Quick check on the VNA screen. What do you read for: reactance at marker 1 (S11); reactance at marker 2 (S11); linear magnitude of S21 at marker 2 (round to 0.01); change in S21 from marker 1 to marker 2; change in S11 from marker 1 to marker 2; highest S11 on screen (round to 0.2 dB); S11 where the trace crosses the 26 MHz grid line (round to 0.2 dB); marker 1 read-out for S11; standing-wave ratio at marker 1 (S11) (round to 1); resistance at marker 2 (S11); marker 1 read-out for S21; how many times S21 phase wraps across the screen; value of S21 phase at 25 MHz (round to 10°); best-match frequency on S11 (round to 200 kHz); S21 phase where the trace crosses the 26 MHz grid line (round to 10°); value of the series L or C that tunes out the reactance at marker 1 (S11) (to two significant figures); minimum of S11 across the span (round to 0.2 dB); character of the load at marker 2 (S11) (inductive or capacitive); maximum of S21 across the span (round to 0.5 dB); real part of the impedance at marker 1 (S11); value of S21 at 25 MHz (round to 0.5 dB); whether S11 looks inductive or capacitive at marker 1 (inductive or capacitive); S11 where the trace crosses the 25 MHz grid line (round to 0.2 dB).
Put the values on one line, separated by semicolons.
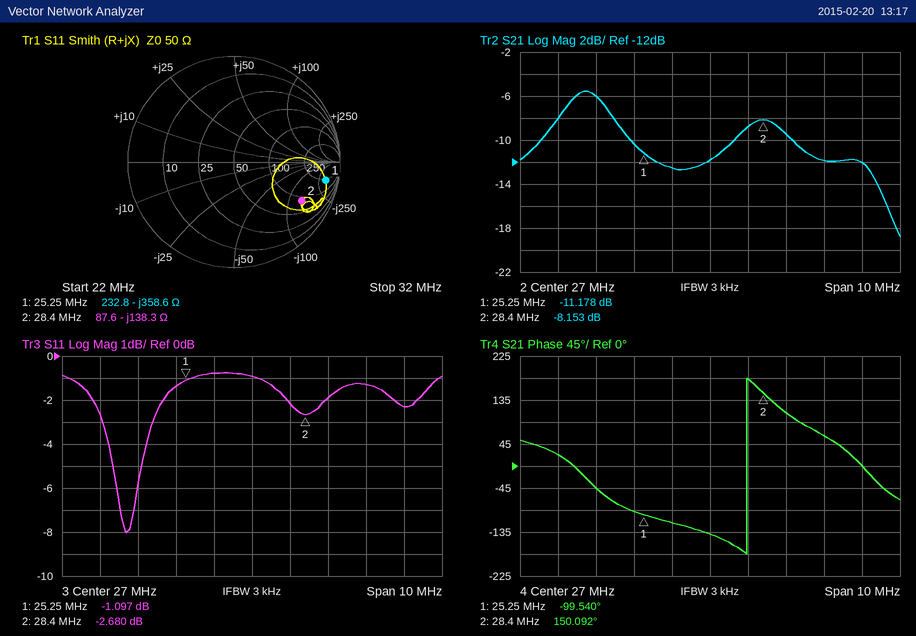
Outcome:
-358.6 Ω; -138.3 Ω; 0.39; 3.025 dB; -1.583 dB; -0.8 dB; -0.8 dB; -1.097 dB; 16; 87.6 Ω; -11.178 dB; 1; -90°; 23.6 MHz; -120°; 2.3 µH; -8.0 dB; capacitive; -5.5 dB; 232.8 Ω; -10.5 dB; capacitive; -1.4 dB
